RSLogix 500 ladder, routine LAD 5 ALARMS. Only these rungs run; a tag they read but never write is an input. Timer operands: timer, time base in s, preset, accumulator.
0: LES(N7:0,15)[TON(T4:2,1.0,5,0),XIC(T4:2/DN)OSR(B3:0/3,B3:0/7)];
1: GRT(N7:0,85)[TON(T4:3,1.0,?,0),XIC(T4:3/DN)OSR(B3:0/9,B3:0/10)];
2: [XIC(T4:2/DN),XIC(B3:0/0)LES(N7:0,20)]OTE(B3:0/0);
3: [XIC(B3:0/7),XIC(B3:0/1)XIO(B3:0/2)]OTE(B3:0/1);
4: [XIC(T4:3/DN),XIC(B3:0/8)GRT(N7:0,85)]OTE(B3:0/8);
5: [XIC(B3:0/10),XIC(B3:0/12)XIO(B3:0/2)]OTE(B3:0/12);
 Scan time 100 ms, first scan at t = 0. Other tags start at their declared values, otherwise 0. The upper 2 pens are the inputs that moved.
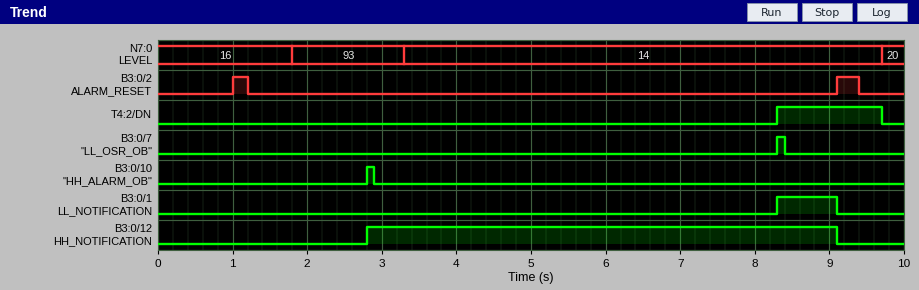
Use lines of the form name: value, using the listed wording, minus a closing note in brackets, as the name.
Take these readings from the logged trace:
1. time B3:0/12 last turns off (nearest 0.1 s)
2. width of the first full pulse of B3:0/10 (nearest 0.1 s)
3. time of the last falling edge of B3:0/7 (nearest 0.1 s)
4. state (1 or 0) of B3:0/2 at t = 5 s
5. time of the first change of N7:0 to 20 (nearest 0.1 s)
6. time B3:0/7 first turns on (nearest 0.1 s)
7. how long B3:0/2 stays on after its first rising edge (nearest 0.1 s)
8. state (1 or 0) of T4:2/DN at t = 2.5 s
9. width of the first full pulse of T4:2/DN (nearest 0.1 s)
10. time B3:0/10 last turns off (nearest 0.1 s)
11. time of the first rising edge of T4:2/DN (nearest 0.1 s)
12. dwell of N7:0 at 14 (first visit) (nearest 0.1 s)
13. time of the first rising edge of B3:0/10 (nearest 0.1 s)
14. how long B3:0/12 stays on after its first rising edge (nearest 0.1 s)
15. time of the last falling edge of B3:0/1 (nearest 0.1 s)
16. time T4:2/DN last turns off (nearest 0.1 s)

time B3:0/12 last turns off: 9.1 s
width of the first full pulse of B3:0/10: 0.1 s
time of the last falling edge of B3:0/7: 8.4 s
state (1 or 0) of B3:0/2 at t = 5 s: 0
time of the first change of N7:0 to 20: 9.7 s
time B3:0/7 first turns on: 8.3 s
how long B3:0/2 stays on after its first rising edge: 0.2 s
state (1 or 0) of T4:2/DN at t = 2.5 s: 0
width of the first full pulse of T4:2/DN: 1.4 s
time B3:0/10 last turns off: 2.9 s
time of the first rising edge of T4:2/DN: 8.3 s
dwell of N7:0 at 14 (first visit): 6.4 s
time of the first rising edge of B3:0/10: 2.8 s
how long B3:0/12 stays on after its first rising edge: 6.3 s
time of the last falling edge of B3:0/1: 9.1 s
time T4:2/DN last turns off: 9.7 s
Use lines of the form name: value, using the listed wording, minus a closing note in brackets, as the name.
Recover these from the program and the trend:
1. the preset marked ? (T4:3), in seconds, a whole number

the preset marked ? (T4:3), in seconds, a whole number: 1 s
